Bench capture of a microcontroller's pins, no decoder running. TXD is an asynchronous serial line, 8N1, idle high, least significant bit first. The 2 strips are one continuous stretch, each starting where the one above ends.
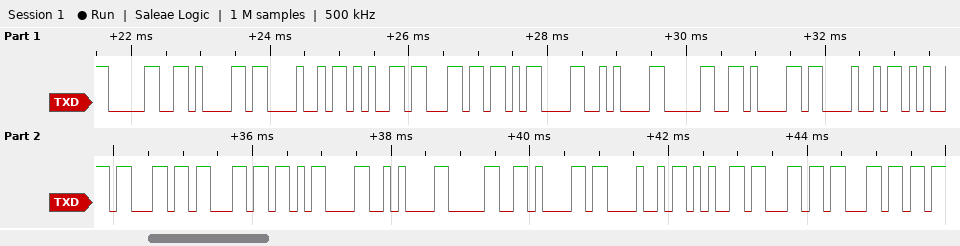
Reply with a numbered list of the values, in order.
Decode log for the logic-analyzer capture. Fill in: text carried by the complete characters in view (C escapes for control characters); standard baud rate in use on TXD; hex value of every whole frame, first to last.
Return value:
1. "0aHel\r\n0aHell\r\n0aHell"
2. 9600 baud
3. 30 61 48 65 6C 0D 0A 30 61 48 65 6C 6C 0D 0A 30 61 48 65 6C 6C
